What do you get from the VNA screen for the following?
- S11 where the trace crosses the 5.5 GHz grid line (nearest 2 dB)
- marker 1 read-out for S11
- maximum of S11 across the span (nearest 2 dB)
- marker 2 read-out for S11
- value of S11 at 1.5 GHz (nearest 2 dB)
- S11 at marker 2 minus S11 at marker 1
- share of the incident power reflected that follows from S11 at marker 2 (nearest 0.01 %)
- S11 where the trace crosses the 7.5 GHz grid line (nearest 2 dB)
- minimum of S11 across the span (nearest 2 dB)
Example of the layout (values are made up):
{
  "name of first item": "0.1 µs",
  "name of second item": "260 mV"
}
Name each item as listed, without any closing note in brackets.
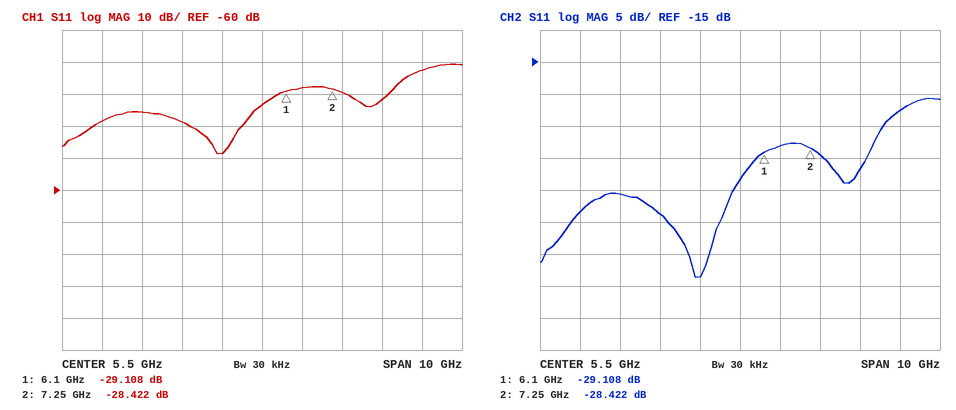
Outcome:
{
  "S11 where the trace crosses the 5.5 GHz grid line": "-34 dB",
  "marker 1 read-out for S11": "-29.108 dB",
  "maximum of S11 across the span": "-20 dB",
  "marker 2 read-out for S11": "-28.422 dB",
  "value of S11 at 1.5 GHz": "-38 dB",
  "S11 at marker 2 minus S11 at marker 1": "0.686 dB",
  "share of the incident power reflected that follows from S11 at marker 2": "0.14 %",
  "S11 where the trace crosses the 7.5 GHz grid line": "-30 dB",
  "minimum of S11 across the span": "-48 dB"
}
